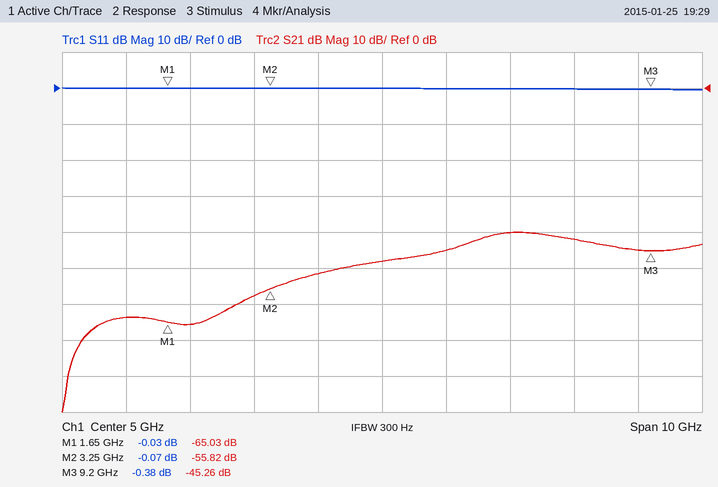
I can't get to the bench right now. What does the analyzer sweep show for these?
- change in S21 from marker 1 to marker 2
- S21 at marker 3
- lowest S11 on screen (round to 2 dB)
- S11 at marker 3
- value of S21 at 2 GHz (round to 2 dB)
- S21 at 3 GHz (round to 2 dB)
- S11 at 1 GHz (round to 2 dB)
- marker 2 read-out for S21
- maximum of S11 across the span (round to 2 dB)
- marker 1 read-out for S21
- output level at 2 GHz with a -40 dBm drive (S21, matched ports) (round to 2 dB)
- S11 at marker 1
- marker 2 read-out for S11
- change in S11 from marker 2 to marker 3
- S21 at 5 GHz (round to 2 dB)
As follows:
9.21 dB
-45.26 dB
0 dB
-0.38 dB
-66 dB
-58 dB
0 dB
-55.82 dB
0 dB
-65.03 dB
-106 dBm
-0.03 dB
-0.07 dB
-0.31 dB
-48 dB
